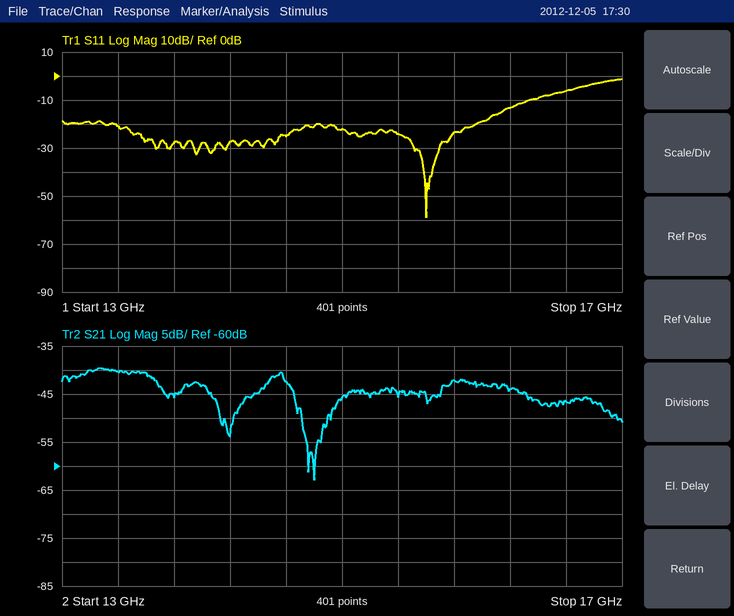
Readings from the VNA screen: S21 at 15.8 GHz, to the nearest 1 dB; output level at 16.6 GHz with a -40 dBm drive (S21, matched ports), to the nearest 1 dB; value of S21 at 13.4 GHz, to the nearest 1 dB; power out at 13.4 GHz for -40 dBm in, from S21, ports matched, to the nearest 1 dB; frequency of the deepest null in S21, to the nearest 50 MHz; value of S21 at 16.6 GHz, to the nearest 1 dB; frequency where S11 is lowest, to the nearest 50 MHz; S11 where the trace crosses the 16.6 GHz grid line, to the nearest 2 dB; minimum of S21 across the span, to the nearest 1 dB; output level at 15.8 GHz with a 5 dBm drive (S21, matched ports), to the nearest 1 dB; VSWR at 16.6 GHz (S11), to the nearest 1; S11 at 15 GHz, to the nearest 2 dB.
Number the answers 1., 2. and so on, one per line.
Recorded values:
1. -42 dB
2. -87 dBm
3. -40 dB
4. -80 dBm
5. 14.80 GHz
6. -47 dB
7. 15.60 GHz
8. -6 dB
9. -63 dB
10. -37 dBm
11. 3
12. -22 dB
